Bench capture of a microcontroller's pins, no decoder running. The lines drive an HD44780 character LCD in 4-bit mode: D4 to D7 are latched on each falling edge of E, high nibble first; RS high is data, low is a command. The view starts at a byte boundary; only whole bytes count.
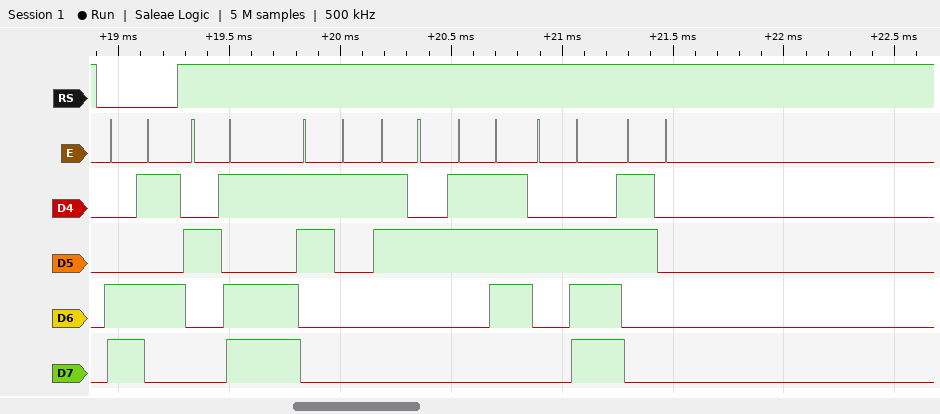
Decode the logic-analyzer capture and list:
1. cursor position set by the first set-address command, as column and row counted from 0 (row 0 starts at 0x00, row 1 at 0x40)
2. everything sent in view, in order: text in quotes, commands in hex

column 5, row 1
0xC5 "-127.0"
